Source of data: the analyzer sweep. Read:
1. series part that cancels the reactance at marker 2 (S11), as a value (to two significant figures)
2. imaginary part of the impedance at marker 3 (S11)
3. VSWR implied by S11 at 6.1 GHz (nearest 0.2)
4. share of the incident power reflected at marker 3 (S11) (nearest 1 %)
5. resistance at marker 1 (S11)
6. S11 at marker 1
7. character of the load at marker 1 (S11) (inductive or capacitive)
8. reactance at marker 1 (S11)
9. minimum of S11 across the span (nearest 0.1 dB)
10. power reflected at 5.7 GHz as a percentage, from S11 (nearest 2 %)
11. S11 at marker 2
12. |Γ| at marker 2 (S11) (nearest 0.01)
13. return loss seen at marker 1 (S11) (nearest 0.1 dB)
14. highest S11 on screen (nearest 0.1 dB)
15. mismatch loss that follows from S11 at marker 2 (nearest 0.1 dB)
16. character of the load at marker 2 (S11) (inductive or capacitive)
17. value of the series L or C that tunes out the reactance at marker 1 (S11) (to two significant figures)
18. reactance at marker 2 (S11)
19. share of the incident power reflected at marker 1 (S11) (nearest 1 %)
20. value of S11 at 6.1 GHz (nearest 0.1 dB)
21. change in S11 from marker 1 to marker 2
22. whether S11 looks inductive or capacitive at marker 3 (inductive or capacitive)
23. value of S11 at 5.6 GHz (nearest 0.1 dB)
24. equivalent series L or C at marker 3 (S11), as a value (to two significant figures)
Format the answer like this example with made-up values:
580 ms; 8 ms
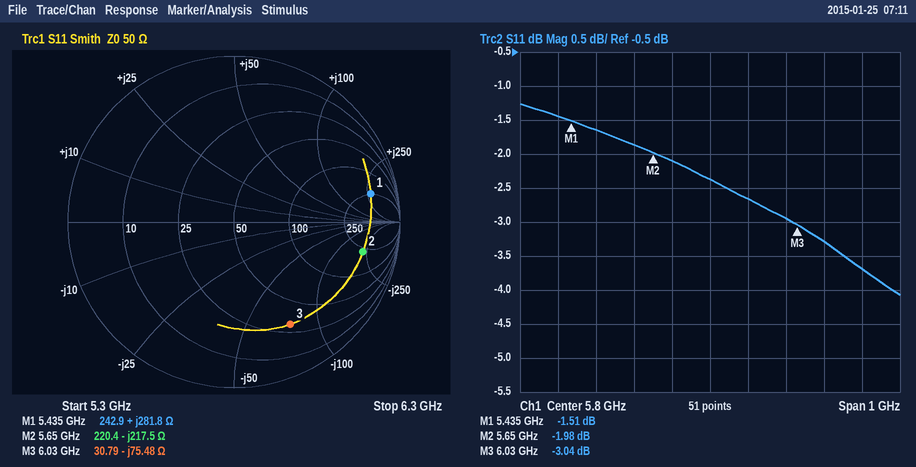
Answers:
6.1 nH; -75.48 Ω; 5.4; 50 %; 242.9 Ω; -1.51 dB; inductive; +281.8 Ω; -4.1 dB; 62 %; -1.98 dB; 0.80; 1.5 dB; -1.3 dB; 4.4 dB; capacitive; 100 fF; -217.5 Ω; 71 %; -3.3 dB; -0.47 dB; capacitive; -1.9 dB; 350 fF
